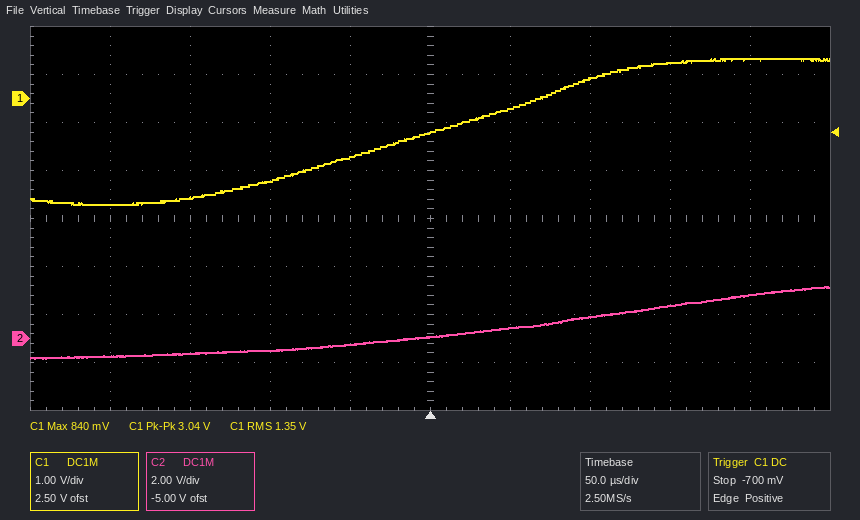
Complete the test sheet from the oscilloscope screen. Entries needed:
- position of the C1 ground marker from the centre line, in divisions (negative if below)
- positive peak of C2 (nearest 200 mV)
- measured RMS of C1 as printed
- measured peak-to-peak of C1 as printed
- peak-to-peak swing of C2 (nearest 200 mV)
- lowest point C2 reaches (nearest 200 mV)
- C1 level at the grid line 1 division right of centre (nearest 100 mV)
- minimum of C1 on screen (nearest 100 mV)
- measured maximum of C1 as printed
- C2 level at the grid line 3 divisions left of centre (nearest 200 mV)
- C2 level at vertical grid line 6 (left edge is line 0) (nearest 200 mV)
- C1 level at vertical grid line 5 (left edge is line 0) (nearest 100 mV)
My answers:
+2.5 div
2.2 V
1.35 V
3.04 V
3.0 V
-800 mV
-200 mV
-2.2 V
840 mV
-600 mV
400 mV
-700 mV
